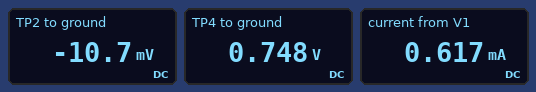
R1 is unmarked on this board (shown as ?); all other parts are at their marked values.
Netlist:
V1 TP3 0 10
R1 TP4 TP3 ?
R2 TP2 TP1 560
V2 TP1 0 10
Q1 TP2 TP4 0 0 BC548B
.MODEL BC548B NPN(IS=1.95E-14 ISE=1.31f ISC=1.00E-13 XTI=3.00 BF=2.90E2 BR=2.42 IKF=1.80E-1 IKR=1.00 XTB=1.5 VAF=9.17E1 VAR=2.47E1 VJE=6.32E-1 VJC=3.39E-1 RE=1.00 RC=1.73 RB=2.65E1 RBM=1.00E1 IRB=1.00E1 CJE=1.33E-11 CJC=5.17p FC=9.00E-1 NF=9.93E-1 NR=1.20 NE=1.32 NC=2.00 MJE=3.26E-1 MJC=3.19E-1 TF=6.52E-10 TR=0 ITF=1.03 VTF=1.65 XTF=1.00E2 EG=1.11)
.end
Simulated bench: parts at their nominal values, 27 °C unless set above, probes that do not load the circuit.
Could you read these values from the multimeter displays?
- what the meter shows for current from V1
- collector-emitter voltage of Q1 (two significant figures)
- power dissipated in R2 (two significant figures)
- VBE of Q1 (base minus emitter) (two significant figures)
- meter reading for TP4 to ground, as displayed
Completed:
0.617 mA
-11 mV
180 mW
750 mV
0.748 V
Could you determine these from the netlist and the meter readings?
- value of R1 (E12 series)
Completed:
15 kΩ
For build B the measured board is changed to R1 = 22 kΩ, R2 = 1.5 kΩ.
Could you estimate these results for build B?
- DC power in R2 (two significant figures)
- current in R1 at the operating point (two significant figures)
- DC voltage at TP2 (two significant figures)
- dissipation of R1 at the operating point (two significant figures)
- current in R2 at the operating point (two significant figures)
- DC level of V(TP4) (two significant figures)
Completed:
67 mW
420 µA
-56 mV
3.9 mW
6.7 mA
710 mV
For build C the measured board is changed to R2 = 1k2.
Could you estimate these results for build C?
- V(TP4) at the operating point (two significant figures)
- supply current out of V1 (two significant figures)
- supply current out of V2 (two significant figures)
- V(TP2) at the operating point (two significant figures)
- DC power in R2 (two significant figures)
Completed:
720 mV
620 µA
8.4 mA
-57 mV
84 mW
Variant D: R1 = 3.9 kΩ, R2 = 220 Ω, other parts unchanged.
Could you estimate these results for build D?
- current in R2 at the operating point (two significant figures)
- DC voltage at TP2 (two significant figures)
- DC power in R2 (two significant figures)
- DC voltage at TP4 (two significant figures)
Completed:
45 mA
52 mV
450 mW
850 mV
